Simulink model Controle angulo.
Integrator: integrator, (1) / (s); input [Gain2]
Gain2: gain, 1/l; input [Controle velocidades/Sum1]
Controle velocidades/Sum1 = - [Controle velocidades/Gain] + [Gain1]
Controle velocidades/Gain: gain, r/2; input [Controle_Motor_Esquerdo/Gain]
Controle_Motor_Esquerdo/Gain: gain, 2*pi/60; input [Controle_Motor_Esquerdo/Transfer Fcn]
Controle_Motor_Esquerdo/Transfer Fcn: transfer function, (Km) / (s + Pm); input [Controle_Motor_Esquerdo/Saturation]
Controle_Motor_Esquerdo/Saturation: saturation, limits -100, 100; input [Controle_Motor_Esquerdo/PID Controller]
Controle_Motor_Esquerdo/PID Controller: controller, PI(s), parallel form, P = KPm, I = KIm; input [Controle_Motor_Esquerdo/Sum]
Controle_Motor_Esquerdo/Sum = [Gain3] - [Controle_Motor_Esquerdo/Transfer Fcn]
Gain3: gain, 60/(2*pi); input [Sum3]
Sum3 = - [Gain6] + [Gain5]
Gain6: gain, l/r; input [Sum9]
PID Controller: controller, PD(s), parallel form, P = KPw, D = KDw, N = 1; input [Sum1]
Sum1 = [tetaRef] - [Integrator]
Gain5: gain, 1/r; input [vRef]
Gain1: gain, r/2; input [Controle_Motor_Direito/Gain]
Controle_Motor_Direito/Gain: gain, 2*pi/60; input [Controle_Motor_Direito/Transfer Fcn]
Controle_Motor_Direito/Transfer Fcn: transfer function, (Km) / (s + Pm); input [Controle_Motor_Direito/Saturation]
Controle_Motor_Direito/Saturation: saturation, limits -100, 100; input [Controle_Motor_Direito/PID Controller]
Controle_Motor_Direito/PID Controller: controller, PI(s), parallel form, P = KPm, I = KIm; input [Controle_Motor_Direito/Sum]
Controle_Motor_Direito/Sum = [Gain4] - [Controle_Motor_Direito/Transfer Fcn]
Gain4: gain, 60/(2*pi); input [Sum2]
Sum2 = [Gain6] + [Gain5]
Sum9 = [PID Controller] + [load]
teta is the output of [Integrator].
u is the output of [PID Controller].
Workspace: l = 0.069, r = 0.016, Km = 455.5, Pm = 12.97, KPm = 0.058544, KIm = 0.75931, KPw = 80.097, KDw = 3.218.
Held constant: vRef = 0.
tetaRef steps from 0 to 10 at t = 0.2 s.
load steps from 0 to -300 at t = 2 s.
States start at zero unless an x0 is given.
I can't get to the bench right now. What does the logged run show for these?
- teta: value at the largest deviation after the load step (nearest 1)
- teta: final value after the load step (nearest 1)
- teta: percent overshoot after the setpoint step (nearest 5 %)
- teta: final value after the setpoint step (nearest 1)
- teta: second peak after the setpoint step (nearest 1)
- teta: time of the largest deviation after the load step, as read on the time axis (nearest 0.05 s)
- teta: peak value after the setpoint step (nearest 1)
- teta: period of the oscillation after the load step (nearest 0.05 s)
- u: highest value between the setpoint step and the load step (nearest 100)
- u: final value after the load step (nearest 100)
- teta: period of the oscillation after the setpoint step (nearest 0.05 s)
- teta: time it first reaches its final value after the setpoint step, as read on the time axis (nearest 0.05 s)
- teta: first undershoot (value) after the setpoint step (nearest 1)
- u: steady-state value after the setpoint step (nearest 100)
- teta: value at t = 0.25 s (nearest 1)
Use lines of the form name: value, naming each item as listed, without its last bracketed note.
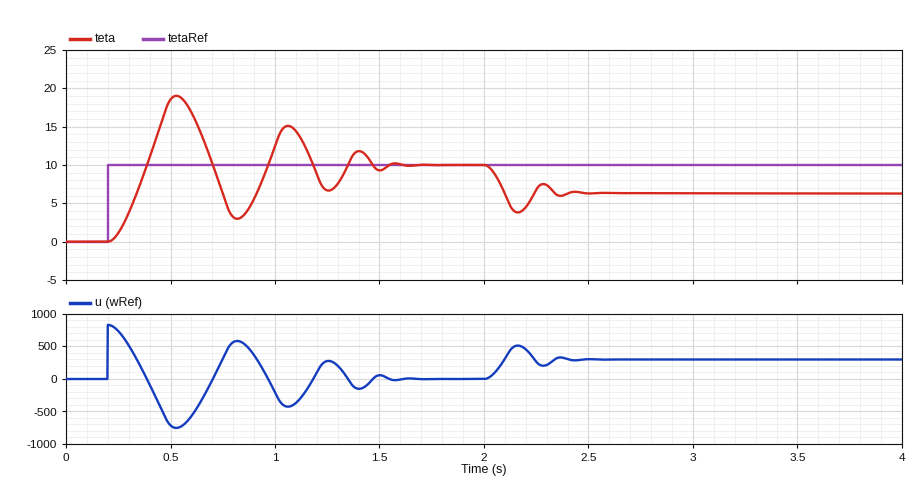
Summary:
teta: value at the largest deviation after the load step: 4
teta: final value after the load step: 6
teta: percent overshoot after the setpoint step: 90 %
teta: final value after the setpoint step: 10
teta: second peak after the setpoint step: 15
teta: time of the largest deviation after the load step, as read on the time axis: 2.15 s
teta: peak value after the setpoint step: 19
teta: period of the oscillation after the load step: 0.20 s
u: highest value between the setpoint step and the load step: 800
u: final value after the load step: 300
teta: period of the oscillation after the setpoint step: 0.55 s
teta: time it first reaches its final value after the setpoint step, as read on the time axis: 0.40 s
teta: first undershoot (value) after the setpoint step: 3
u: steady-state value after the setpoint step: 0
teta: value at t = 0.25 s: 1
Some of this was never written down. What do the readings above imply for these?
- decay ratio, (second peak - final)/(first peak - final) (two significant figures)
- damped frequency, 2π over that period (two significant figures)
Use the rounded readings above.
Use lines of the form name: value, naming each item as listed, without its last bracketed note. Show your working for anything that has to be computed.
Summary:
decay ratio, (second peak - final)/(first peak - final): (15 - 10) / (19 - 10) = 0.56
damped frequency, 2π over that period: 2π / 0.55 = 11 rad/s
